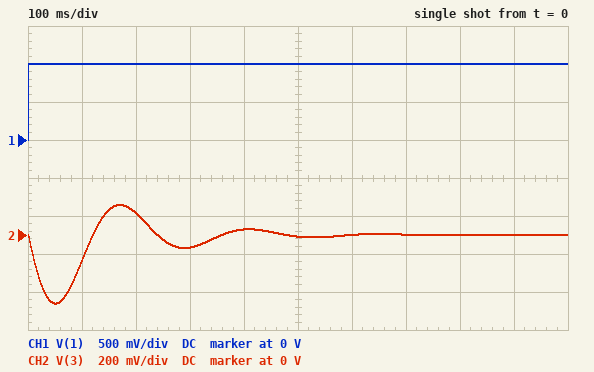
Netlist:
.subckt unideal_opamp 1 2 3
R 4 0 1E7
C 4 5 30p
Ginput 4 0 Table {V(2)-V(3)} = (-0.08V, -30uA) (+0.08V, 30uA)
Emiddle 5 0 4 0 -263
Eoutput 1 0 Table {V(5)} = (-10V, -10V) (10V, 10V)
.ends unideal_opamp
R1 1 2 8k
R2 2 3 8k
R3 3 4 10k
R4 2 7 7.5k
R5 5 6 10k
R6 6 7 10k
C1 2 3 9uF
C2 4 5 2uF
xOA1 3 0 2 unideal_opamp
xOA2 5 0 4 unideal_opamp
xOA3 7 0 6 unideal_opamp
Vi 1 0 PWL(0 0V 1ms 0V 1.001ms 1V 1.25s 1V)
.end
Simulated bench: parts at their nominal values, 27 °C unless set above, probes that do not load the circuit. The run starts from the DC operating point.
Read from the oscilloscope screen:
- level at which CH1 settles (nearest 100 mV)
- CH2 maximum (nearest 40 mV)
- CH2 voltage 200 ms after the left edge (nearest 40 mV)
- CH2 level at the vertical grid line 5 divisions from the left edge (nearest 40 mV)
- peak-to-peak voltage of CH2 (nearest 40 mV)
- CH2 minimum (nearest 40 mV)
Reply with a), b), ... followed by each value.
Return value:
a) 1.0 V
b) 160 mV
c) 120 mV
d) 0 V
e) 520 mV
f) -360 mV
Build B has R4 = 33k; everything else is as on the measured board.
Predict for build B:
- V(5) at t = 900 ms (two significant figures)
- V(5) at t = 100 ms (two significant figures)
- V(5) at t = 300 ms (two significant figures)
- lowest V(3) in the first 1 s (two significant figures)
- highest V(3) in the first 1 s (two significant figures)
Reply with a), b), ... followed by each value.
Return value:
a) 4.1 V
b) 2.0 V
c) 4.7 V
d) -570 mV
e) 77 mV
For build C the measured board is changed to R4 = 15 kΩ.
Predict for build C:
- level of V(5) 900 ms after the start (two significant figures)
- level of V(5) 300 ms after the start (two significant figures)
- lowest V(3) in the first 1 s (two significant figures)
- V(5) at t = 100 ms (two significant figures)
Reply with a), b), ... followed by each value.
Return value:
a) 1.9 V
b) 1.8 V
c) -450 mV
d) 1.7 V
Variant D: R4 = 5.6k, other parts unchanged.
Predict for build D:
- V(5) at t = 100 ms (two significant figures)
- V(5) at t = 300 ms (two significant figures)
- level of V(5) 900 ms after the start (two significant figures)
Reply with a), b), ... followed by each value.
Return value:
a) 1.0 V
b) 780 mV
c) 700 mV
